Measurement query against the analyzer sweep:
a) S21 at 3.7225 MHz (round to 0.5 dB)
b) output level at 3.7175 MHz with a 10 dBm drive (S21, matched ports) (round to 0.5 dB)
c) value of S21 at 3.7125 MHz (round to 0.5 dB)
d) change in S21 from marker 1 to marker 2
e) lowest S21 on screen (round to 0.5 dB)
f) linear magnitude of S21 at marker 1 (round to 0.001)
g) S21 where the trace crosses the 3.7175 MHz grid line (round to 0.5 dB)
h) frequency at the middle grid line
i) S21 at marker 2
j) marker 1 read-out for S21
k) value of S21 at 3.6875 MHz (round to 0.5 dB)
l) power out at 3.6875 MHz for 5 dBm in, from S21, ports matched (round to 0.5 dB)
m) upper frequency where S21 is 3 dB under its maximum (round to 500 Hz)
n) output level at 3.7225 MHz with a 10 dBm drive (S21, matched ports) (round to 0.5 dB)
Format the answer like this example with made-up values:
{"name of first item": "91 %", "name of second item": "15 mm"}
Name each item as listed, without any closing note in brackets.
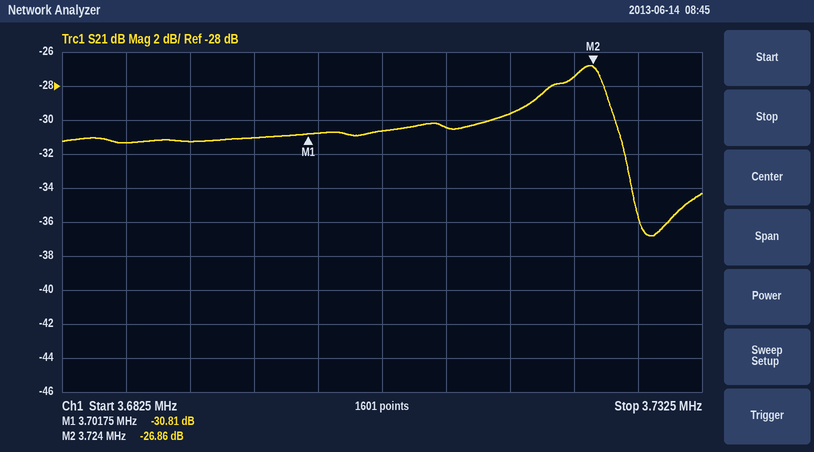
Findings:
{"S21 at 3.7225 MHz": "-27.5 dB", "output level at 3.7175 MHz with a 10 dBm drive (S21, matched ports)": "-19.5 dBm", "value of S21 at 3.7125 MHz": "-30.5 dB", "change in S21 from marker 1 to marker 2": "3.95 dB", "lowest S21 on screen": "-37.0 dB", "linear magnitude of S21 at marker 1": "0.029", "S21 where the trace crosses the 3.7175 MHz grid line": "-29.5 dB", "frequency at the middle grid line": "3.7075 MHz", "S21 at marker 2": "-26.86 dB", "marker 1 read-out for S21": "-30.81 dB", "value of S21 at 3.6875 MHz": "-31.5 dB", "power out at 3.6875 MHz for 5 dBm in, from S21, ports matched": "-26.5 dBm", "upper frequency where S21 is 3 dB under its maximum": "3.7255 MHz", "output level at 3.7225 MHz with a 10 dBm drive (S21, matched ports)": "-17.5 dBm"}
